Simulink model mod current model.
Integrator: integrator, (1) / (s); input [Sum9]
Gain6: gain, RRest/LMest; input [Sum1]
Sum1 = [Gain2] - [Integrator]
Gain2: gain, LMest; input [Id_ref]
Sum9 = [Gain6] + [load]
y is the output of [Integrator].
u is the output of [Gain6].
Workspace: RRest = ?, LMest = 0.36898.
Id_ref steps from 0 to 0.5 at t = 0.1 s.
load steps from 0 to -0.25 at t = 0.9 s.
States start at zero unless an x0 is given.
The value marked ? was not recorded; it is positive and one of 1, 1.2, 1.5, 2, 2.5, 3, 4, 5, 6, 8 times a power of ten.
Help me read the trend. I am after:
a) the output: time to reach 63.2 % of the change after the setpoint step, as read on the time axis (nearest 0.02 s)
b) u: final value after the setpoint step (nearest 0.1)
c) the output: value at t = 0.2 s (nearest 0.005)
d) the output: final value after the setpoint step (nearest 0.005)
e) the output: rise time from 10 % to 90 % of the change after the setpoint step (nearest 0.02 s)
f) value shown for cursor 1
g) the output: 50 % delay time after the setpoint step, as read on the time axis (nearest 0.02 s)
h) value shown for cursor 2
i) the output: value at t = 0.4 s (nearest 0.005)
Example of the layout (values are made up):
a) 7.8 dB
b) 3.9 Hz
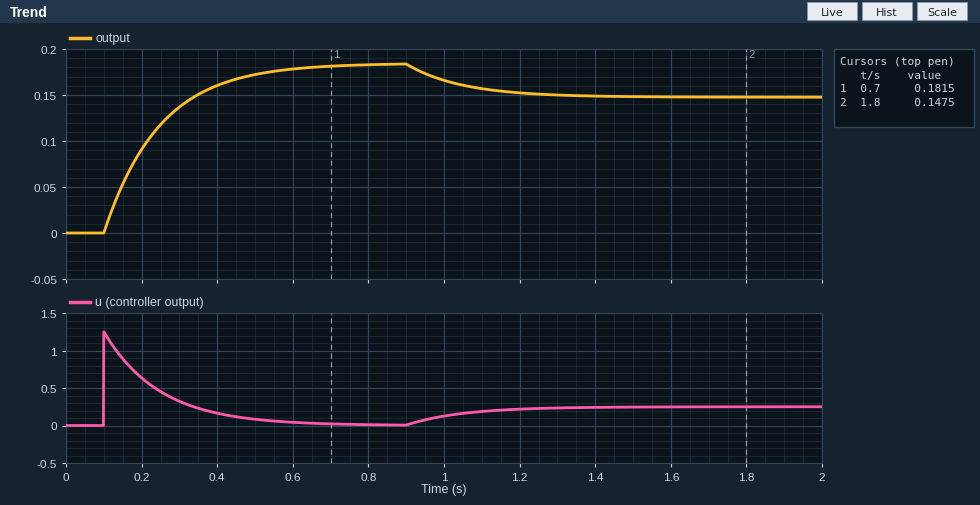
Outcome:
a) 0.24 s
b) 0.0
c) 0.090
d) 0.185
e) 0.32 s
f) 0.1815
g) 0.20 s
h) 0.1475
i) 0.160
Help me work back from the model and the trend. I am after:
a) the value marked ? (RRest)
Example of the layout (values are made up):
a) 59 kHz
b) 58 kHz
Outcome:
a) 2.5
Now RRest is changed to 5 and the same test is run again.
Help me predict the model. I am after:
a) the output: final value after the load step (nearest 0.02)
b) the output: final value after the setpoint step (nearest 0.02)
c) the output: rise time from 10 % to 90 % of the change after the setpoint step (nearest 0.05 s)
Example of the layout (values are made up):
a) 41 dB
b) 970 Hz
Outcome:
a) 0.16
b) 0.18
c) 0.15 s
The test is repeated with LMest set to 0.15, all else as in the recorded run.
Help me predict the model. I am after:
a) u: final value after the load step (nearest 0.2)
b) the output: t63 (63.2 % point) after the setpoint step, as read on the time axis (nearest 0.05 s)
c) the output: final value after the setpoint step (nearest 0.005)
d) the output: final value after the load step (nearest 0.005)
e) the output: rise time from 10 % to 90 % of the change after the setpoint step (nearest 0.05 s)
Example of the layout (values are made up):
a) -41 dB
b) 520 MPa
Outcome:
a) 0.2
b) 0.15 s
c) 0.075
d) 0.060
e) 0.15 s
